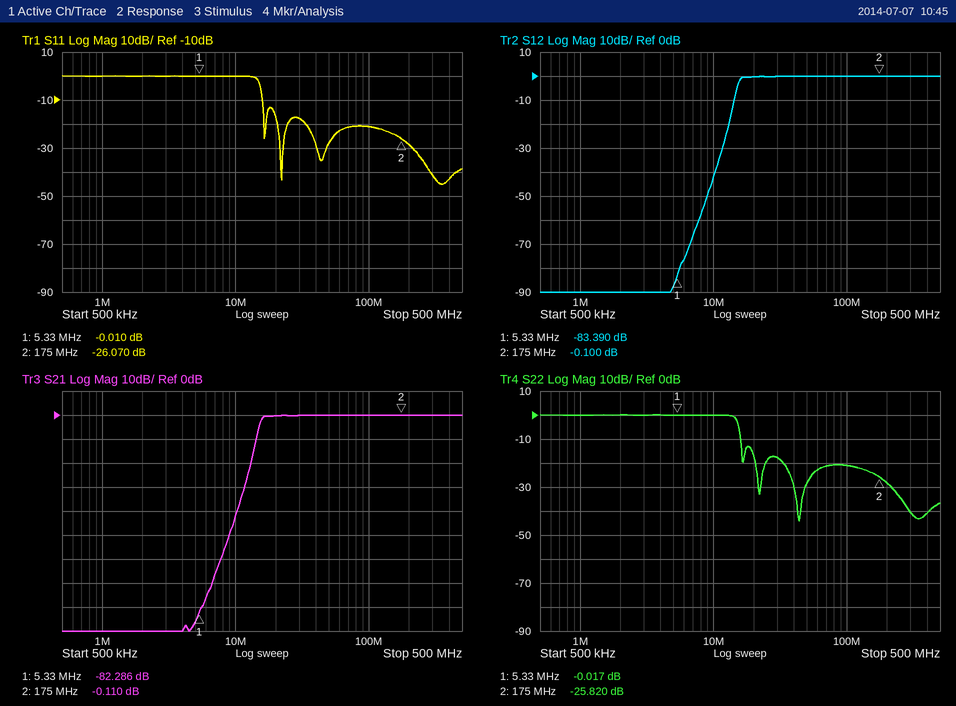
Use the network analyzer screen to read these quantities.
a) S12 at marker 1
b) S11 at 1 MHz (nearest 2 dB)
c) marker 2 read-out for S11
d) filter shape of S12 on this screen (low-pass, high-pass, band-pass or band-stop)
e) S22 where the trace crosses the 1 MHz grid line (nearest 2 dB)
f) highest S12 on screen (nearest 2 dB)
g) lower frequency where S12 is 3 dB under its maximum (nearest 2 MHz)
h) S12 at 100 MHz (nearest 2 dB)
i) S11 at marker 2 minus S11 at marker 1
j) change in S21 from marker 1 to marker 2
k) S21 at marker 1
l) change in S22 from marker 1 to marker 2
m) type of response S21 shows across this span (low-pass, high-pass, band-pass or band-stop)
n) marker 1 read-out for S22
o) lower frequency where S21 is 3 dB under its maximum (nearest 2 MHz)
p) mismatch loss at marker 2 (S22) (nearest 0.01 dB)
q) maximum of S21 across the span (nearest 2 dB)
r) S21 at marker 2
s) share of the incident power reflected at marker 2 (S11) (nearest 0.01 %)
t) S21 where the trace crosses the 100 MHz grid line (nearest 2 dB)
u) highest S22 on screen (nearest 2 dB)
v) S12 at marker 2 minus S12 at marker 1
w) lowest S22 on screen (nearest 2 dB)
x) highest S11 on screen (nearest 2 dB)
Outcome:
-83.390 dB
0 dB
-26.070 dB
high-pass
0 dB
0 dB
16 MHz
0 dB
-26.060 dB
82.176 dB
-82.286 dB
-25.803 dB
high-pass
-0.017 dB
16 MHz
0.01 dB
0 dB
-0.110 dB
0.25 %
0 dB
0 dB
83.290 dB
-44 dB
0 dB
